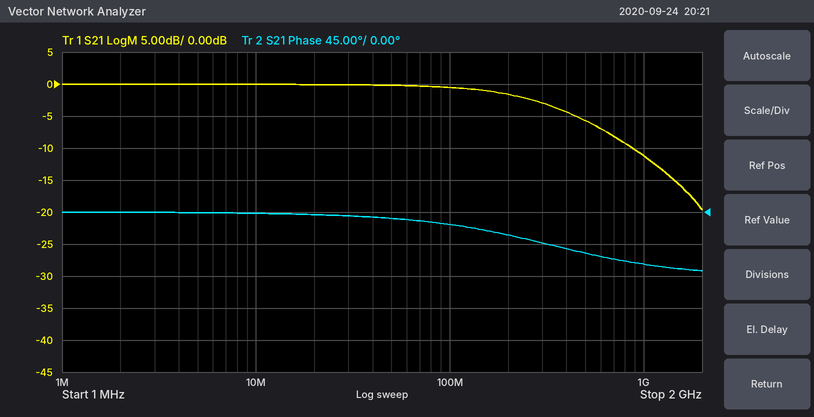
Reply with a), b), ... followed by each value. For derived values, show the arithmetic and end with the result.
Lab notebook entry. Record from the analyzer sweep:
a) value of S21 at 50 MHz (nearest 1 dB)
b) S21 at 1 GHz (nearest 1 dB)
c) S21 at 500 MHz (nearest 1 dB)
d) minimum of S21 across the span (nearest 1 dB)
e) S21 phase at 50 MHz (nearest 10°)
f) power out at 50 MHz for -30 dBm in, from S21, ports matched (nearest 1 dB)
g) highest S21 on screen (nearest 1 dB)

a) 0 dB
b) -11 dB
c) -6 dB
d) -20 dB
e) -10°
f) -30 dBm + (0 dB) = -30 dBm
g) 0 dB
